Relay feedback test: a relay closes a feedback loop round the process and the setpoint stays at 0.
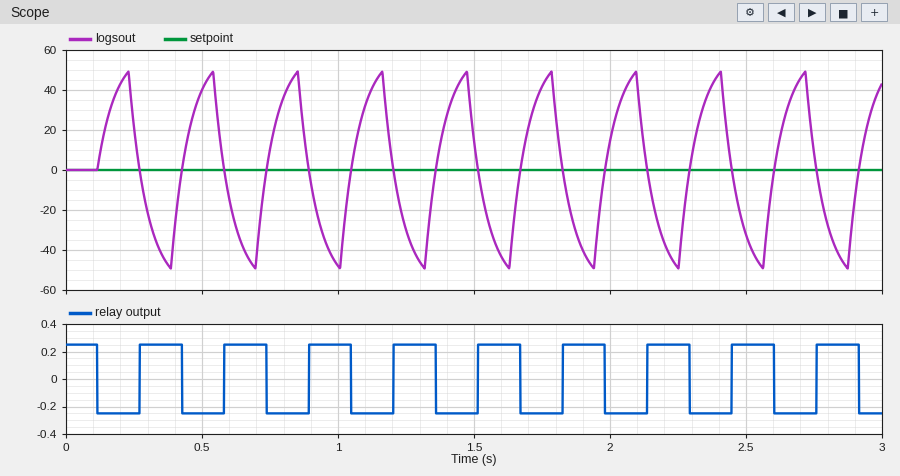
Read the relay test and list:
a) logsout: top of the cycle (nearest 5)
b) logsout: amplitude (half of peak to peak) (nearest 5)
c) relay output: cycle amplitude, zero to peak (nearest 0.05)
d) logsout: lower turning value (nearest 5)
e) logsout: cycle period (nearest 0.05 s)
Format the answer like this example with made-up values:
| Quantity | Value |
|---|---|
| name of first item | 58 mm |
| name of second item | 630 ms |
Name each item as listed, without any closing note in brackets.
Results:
| Quantity | Value |
|---|---|
| logsout: top of the cycle | 50 |
| logsout: amplitude (half of peak to peak) | 50 |
| relay output: cycle amplitude, zero to peak | 0.25 |
| logsout: lower turning value | -50 |
| logsout: cycle period | 0.30 s |
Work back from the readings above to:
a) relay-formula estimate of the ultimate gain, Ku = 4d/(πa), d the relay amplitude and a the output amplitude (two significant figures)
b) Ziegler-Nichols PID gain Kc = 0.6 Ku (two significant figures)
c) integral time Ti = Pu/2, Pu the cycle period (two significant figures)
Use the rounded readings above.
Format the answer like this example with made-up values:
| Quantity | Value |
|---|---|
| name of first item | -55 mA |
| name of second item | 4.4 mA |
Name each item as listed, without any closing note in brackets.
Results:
| Quantity | Value |
|---|---|
| relay-formula estimate of the ultimate gain, Ku = 4d/(πa), d the relay amplitude and a the output amplitude | 0.0064 |
| Ziegler-Nichols PID gain Kc = 0.6 Ku | 0.0038 |
| integral time Ti = Pu/2, Pu the cycle period | 0.15 s |
